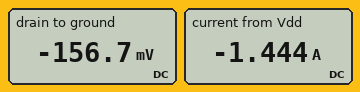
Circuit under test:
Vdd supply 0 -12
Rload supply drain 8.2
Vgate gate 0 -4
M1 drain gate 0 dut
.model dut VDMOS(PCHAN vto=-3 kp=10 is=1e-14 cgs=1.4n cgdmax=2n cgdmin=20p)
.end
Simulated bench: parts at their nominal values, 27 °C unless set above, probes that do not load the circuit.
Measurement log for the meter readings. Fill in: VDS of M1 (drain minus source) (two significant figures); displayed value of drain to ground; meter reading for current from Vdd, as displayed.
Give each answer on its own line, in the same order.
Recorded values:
-160 mV
-156.7 mV
-1.444 A
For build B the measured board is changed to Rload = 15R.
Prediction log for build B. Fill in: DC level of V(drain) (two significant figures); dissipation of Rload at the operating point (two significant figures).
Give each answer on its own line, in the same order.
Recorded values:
-83 mV
9.5 W
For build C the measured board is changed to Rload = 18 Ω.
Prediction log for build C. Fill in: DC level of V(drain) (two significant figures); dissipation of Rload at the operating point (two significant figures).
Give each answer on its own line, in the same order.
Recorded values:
-69 mV
7.9 W
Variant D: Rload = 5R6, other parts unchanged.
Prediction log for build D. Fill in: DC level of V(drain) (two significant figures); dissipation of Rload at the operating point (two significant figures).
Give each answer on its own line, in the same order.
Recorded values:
-240 mV
25 W
